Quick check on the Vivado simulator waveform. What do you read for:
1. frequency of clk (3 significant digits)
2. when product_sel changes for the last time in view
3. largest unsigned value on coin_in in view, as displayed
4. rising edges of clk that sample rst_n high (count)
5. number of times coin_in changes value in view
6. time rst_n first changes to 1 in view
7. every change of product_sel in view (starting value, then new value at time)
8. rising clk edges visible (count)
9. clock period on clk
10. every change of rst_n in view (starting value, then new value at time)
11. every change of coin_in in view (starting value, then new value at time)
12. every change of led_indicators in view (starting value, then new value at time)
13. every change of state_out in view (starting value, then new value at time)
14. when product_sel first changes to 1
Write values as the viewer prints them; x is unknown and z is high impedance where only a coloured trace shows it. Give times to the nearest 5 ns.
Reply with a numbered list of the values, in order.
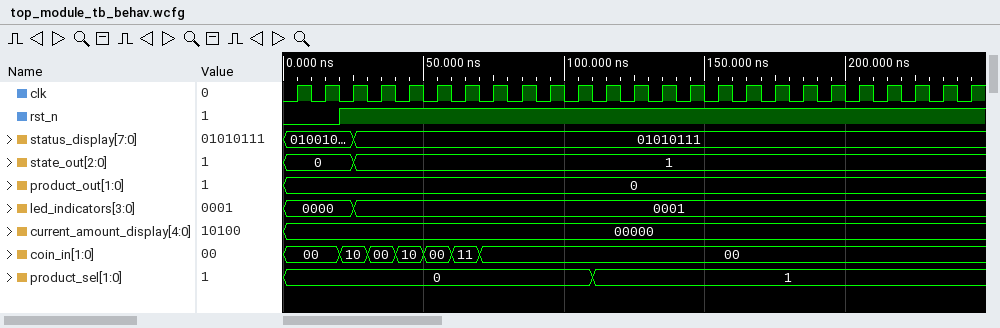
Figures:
1. 100 MHz
2. 110 ns
3. 11
4. 23
5. 6
6. 20 ns
7. 0, 1 at 110 ns
8. 25
9. 10 ns
10. 0, 1 at 20 ns
11. 00, 10 at 20 ns, 00 at 30 ns, 10 at 40 ns, 00 at 50 ns, 11 at 60 ns, 00 at 70 ns
12. 0000, 0001 at 25 ns
13. 0, 1 at 25 ns
14. 110 ns
